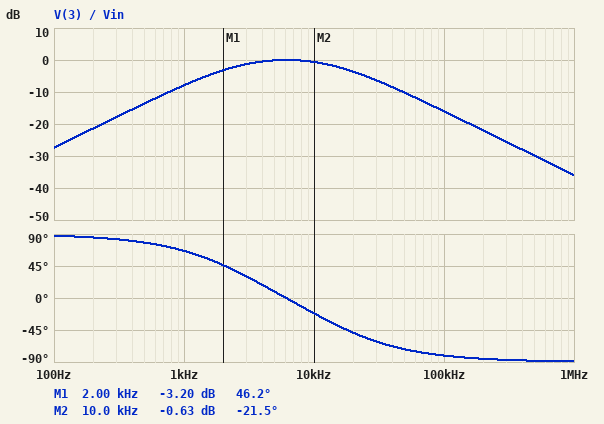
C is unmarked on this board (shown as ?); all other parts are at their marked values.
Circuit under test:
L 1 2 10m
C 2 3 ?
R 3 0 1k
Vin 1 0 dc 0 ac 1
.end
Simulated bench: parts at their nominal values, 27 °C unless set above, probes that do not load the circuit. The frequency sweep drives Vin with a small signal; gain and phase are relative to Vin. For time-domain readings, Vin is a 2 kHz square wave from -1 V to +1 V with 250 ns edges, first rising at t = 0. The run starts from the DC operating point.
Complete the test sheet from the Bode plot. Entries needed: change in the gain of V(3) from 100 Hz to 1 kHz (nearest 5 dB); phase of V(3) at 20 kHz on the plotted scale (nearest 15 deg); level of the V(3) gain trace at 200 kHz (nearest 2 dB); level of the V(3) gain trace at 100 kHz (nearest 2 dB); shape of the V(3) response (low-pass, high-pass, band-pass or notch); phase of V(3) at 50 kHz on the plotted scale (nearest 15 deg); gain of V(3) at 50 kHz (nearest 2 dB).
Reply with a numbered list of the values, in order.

1. 20 dB
2. -45 deg
3. -22 dB
4. -16 dB
5. band-pass
6. -75 deg
7. -10 dB
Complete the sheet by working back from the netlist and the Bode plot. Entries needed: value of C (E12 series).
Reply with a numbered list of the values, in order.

1. 68 nF
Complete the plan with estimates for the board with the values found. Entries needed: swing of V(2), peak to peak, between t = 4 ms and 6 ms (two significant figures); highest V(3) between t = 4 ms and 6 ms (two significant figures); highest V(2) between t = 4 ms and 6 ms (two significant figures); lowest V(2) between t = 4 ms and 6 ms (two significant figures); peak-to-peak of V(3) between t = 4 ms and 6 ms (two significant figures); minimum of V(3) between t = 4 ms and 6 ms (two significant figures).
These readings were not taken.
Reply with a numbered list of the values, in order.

1. 2.4 V
2. 1.6 V
3. 1.2 V
4. -1.2 V
5. 3.1 V
6. -1.6 V
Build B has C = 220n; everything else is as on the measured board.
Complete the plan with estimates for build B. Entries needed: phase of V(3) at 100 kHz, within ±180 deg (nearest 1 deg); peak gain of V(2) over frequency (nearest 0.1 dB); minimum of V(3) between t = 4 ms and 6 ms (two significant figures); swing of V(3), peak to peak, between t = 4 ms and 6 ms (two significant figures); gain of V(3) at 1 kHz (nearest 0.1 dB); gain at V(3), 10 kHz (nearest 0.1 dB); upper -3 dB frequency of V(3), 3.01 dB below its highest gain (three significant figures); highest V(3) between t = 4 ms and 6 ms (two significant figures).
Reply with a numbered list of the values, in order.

1. -81 deg
2. 0.3 dB
3. -1.4 V
4. 2.7 V
5. -1.6 dB
6. -1.2 dB
7. 16.6 kHz
8. 1.4 V
